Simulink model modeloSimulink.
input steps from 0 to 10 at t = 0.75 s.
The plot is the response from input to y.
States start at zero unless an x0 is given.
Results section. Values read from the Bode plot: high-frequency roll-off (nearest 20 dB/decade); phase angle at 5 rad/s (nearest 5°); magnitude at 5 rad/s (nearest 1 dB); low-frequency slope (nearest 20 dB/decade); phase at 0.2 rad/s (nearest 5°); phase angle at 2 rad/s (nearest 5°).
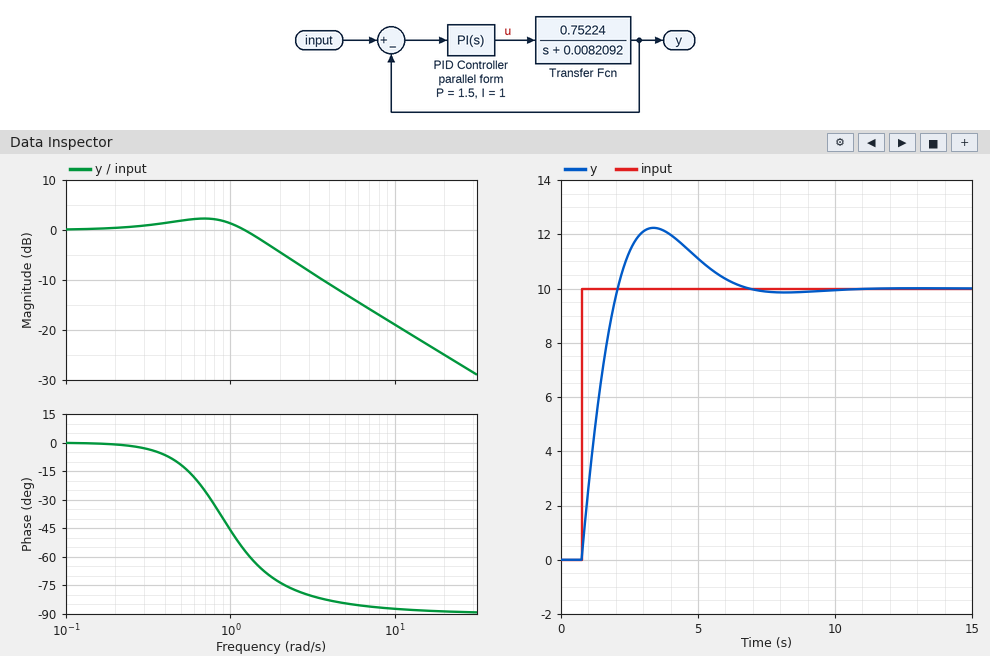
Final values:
-20 dB/decade
-85°
-13 dB
0 dB/decade
0°
-75°
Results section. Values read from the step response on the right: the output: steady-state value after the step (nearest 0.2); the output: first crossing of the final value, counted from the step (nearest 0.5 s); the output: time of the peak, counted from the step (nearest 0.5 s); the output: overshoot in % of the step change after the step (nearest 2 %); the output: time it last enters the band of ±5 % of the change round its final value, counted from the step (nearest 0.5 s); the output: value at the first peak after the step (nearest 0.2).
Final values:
10.0
1.5 s
2.5 s
22 %
5.0 s
12.2
